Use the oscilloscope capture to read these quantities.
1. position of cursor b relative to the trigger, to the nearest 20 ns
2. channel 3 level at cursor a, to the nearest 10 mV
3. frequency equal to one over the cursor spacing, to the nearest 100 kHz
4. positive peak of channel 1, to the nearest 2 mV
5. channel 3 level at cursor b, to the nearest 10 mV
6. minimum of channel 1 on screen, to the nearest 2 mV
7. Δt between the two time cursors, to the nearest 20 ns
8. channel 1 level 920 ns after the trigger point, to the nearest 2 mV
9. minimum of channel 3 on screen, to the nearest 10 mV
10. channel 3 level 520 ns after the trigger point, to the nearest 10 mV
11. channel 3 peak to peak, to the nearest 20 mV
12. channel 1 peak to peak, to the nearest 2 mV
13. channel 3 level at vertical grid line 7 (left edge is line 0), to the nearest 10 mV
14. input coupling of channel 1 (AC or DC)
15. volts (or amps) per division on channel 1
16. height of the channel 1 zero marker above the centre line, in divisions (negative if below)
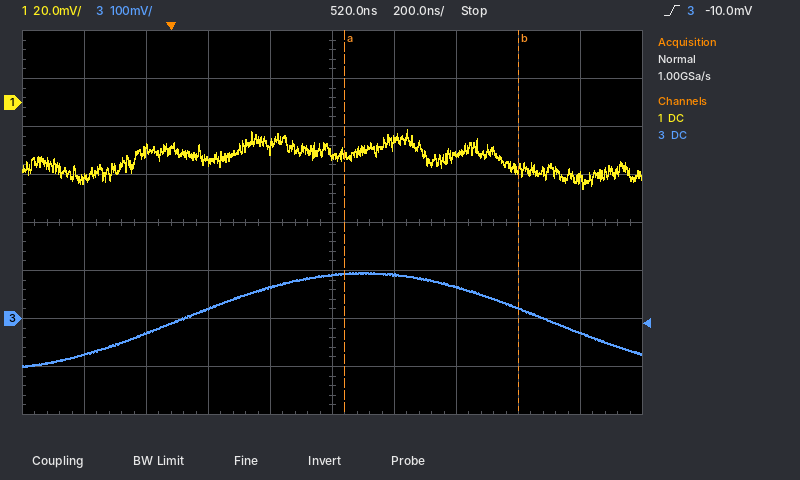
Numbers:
+1.12 µs
90 mV
1.8 MHz
-12 mV
20 mV
-36 mV
560 ns
-22 mV
-100 mV
90 mV
200 mV
24 mV
70 mV
DC
20 mV
+2.5 div
